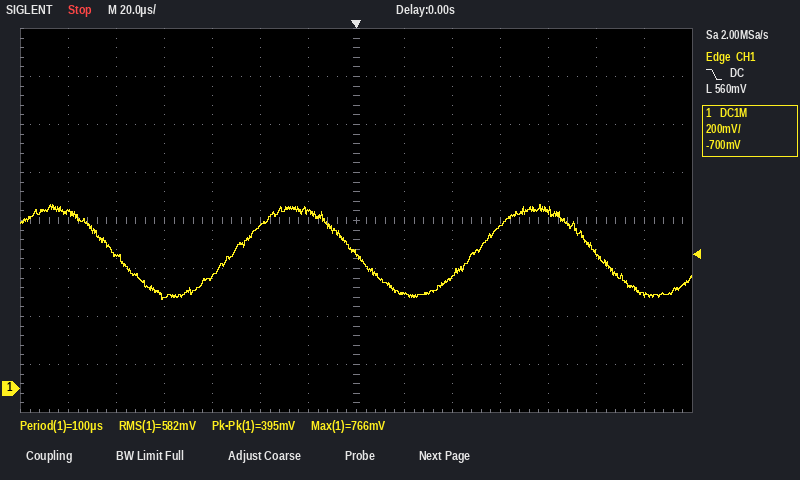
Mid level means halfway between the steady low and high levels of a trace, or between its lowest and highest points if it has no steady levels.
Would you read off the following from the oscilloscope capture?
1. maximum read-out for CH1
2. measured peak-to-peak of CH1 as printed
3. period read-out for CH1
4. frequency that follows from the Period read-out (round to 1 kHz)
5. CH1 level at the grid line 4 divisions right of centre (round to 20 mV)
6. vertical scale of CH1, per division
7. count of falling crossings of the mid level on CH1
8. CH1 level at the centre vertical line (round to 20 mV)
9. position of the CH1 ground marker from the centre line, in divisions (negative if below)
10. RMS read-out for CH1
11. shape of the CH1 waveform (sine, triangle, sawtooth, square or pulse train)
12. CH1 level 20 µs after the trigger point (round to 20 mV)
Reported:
766 mV
395 mV
100 µs
10 kHz
740 mV
200 mV
3
560 mV
-3.5 div
582 mV
sine
400 mV
